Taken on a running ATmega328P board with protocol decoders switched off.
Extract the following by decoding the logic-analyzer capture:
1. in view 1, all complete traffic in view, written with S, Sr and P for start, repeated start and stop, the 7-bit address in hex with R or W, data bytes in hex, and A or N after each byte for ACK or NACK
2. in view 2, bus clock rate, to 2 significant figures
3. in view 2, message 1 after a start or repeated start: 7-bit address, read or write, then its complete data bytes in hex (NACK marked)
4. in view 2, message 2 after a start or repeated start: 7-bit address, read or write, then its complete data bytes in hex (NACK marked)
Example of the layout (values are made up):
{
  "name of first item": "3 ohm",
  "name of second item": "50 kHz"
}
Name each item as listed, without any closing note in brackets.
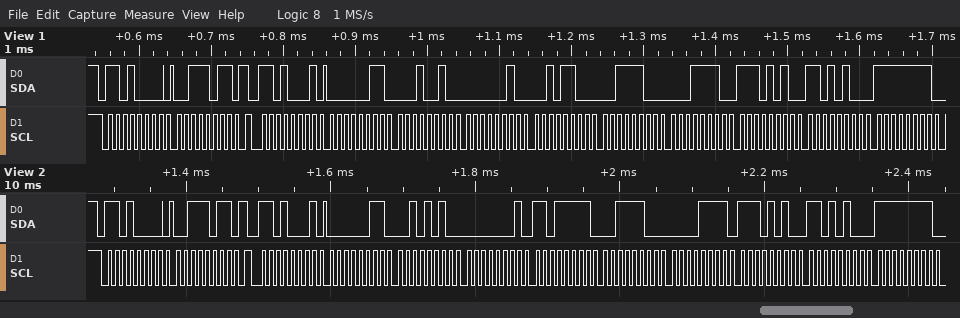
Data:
{
  "in view 1, all complete traffic in view, written with S, Sr and P for start, repeated start and stop, the 7-bit address in hex with R or W, data bytes in hex, and A or N after each byte for ACK or NACK": "S 68W A 3B A Sr 68R A 03 A 12 A 02 A 2C A 3C A 1E A EA A D4 A FF A",
  "in view 2, bus clock rate, to 2 significant figures": "100 kHz",
  "in view 2, message 1 after a start or repeated start: 7-bit address, read or write, then its complete data bytes in hex": "0x68 write: 3B",
  "in view 2, message 2 after a start or repeated start: 7-bit address, read or write, then its complete data bytes in hex": "0x68 read: 03 2A 01 DF 3C 0F EA D4 FF"
}
